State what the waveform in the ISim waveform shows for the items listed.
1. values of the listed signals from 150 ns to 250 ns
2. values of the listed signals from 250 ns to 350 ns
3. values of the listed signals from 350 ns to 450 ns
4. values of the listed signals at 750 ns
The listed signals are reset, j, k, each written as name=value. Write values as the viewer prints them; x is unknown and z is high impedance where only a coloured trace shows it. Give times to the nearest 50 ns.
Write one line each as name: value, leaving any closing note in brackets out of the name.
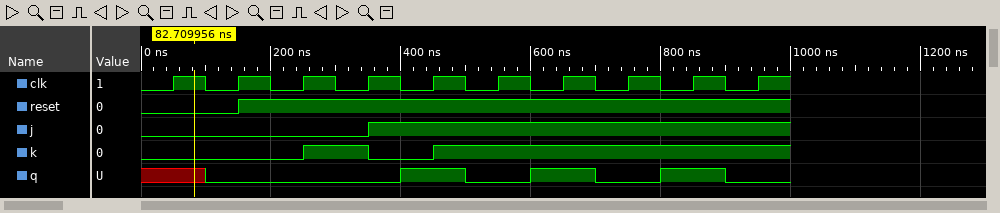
values of the listed signals from 150 ns to 250 ns: reset=1, j=0, k=0
values of the listed signals from 250 ns to 350 ns: reset=1, j=0, k=1
values of the listed signals from 350 ns to 450 ns: reset=1, j=1, k=0
values of the listed signals at 750 ns: reset=1, j=1, k=1
